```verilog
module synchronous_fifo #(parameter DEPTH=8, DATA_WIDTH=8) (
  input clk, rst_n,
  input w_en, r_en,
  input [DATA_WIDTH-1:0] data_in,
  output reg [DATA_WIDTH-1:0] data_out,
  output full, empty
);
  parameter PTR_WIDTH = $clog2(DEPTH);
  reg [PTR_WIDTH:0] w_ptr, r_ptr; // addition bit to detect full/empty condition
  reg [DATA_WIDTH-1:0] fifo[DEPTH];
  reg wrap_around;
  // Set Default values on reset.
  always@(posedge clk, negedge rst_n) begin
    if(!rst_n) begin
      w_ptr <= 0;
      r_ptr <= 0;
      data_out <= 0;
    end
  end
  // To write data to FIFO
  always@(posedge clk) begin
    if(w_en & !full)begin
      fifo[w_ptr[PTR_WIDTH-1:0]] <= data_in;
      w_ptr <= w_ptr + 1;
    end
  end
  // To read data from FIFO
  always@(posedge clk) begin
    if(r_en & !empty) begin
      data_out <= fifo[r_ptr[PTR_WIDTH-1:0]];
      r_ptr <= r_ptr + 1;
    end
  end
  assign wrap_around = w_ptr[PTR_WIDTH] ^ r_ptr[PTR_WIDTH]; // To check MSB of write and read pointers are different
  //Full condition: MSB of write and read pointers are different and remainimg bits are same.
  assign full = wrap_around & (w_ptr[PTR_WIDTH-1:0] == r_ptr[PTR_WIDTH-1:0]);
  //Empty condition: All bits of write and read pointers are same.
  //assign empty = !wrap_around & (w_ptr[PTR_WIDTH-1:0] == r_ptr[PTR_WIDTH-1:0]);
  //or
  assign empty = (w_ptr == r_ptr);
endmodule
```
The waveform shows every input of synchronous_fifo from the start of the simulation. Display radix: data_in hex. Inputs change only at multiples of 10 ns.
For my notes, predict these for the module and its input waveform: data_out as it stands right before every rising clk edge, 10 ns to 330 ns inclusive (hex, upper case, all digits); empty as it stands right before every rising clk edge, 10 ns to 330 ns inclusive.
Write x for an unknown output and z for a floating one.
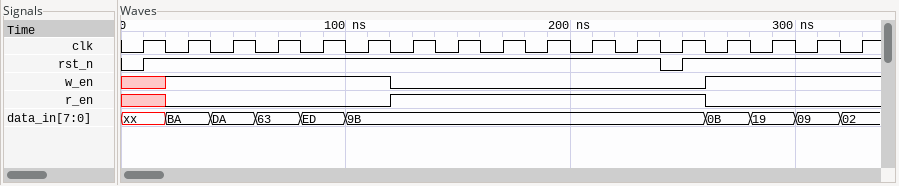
00, 00, 00, 00, 00, 00, 00, BA, DA, 63, ED, 9B, 00, 00, 00, 00, 00
1 1 0 0 0 0 0 0 0 0 0 1 1 1 0 0 0
